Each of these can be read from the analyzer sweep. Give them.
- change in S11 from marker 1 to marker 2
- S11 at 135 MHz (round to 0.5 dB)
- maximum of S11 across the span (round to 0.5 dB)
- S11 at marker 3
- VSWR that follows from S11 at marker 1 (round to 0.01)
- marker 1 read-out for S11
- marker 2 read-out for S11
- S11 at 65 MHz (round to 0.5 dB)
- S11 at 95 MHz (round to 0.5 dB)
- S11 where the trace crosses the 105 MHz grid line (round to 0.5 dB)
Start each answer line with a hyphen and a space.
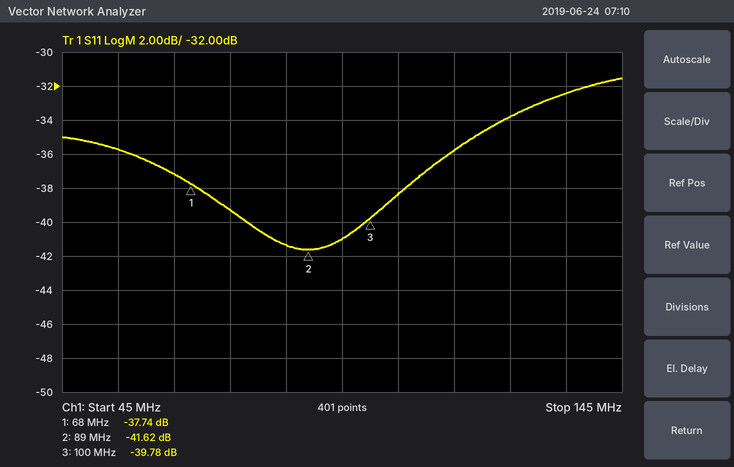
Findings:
- -3.88 dB
- -32.5 dB
- -31.5 dB
- -39.78 dB
- 1.03
- -37.74 dB
- -41.62 dB
- -37.0 dB
- -41.0 dB
- -38.5 dB
